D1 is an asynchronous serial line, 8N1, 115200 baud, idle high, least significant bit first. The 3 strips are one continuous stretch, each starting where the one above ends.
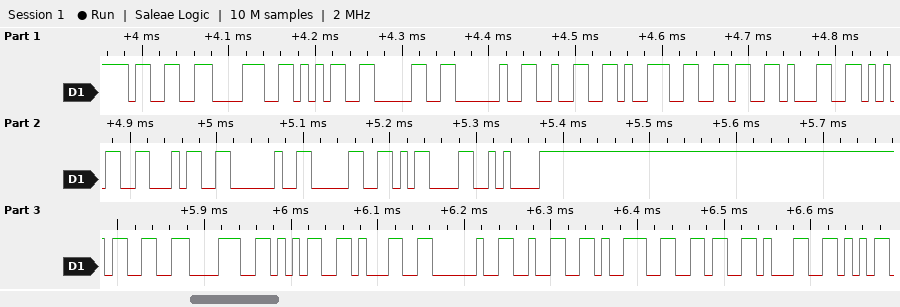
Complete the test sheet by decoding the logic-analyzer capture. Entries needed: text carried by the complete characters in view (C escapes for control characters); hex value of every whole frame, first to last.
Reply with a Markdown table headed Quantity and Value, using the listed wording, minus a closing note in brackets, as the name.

| Quantity | Value |
|---|---|
| text carried by the complete characters in view | "3850 296154 0\r\n3851 2961" |
| hex value of every whole frame, first to last | 33 38 35 30 20 32 39 36 31 35 34 20 30 0D 0A 33 38 35 31 20 32 39 36 31 |
